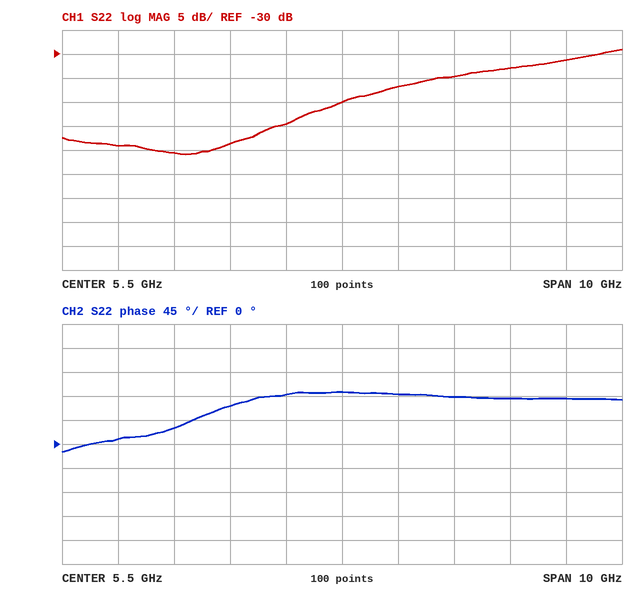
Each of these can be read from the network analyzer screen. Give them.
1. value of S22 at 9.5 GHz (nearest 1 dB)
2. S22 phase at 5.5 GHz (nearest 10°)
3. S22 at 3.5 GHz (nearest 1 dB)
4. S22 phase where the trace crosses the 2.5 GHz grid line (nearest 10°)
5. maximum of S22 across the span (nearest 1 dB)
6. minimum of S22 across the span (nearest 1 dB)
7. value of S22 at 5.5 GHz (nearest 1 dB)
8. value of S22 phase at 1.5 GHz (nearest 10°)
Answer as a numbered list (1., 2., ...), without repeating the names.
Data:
1. -31 dB
2. 100°
3. -49 dB
4. 30°
5. -29 dB
6. -51 dB
7. -40 dB
8. 10°
